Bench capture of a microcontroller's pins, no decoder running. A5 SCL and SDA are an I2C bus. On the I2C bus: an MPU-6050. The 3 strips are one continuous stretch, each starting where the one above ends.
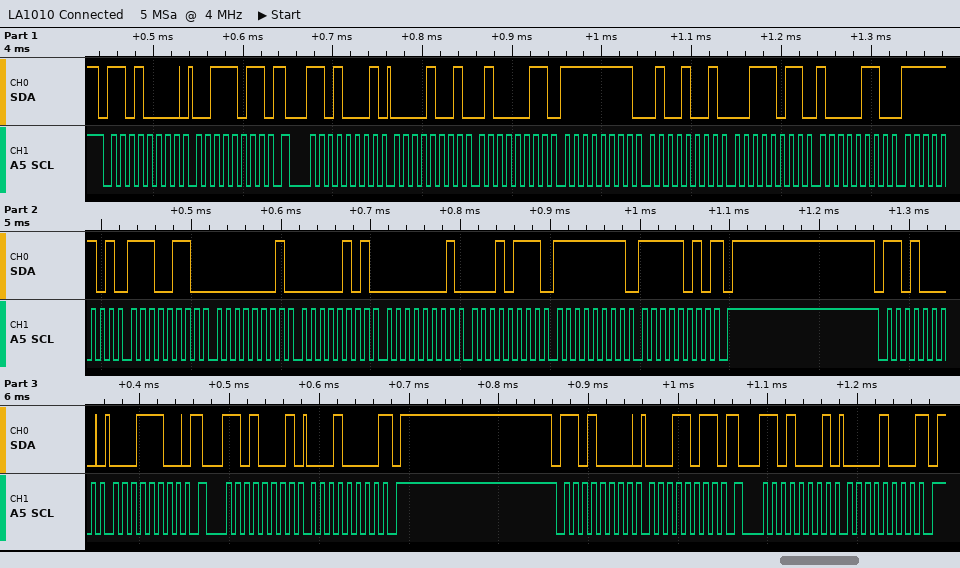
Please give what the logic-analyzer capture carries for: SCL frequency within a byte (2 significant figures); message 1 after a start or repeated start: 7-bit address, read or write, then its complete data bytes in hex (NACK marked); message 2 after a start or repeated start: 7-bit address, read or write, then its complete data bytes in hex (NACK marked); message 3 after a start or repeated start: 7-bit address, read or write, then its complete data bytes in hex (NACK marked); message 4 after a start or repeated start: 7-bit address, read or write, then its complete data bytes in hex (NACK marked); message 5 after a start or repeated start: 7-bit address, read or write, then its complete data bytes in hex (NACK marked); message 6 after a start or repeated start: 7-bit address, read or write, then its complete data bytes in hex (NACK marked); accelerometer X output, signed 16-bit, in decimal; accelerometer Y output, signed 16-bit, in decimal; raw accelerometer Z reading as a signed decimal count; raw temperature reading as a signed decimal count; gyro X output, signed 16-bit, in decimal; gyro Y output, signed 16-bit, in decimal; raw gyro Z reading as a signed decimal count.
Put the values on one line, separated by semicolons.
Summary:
100 kHz; 0x68 write: 3B; 0x68 read: 09 43 FF 49 3B 86 FD E6 01 05 01 17 FF FA NACK; 0x68 write: 1C; 0x68 read: 10 NACK; 0x68 write: 1B; 0x68 read: 08 NACK; 2371; -183; 15238; -538; 261; 279; -6
